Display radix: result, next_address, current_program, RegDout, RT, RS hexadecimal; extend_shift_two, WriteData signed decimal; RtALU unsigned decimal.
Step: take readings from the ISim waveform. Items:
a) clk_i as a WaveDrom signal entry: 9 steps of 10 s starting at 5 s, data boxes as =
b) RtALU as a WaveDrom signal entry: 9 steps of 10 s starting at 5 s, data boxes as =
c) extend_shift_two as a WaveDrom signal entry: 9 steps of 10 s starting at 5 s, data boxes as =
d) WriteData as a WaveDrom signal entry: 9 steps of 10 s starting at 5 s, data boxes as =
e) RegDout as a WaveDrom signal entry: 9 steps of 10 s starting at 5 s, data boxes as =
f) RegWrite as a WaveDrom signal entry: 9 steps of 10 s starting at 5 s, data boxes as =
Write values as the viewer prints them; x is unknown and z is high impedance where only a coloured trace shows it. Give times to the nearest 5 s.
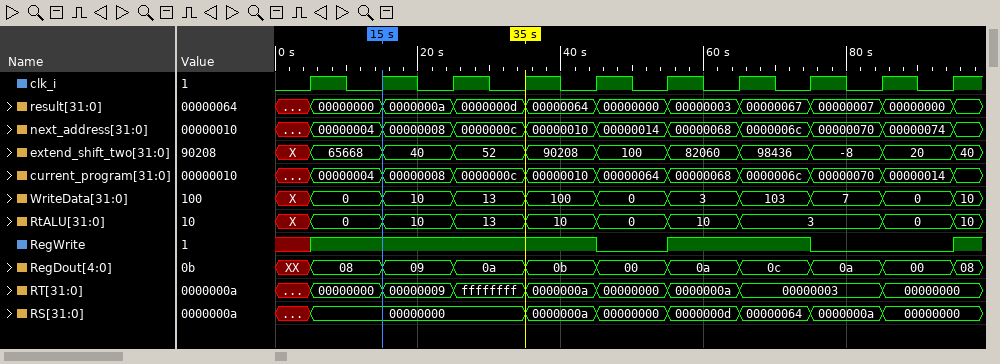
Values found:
{name: 'clk_i', wave: 'p........'}
{name: 'RtALU', wave: '=======.=', data: '0 10 13 10 0 10 3 0'}
{name: 'extend_shift_two', wave: '=========', data: '65668 40 52 90208 100 82060 98436 -8 20'}
{name: 'WriteData', wave: '=========', data: '0 10 13 100 0 3 103 7 0'}
{name: 'RegDout', wave: '=========', data: '08 09 0a 0b 00 0a 0c 0a 00'}
{name: 'RegWrite', wave: '1...01.0.'}
